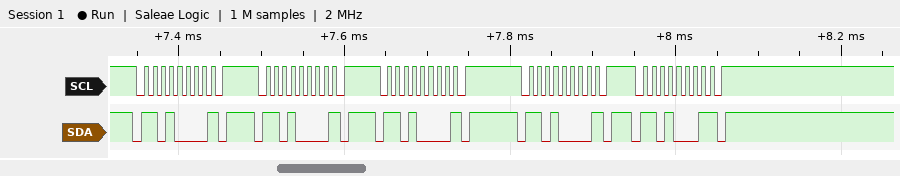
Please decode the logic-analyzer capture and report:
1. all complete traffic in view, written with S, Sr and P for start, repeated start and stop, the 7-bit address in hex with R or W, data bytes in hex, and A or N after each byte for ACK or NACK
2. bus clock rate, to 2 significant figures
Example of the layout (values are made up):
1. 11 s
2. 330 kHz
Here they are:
1. S 68W N P S 68W N P S 68W N P S 68W N P S 68R N P
2. 100 kHz
